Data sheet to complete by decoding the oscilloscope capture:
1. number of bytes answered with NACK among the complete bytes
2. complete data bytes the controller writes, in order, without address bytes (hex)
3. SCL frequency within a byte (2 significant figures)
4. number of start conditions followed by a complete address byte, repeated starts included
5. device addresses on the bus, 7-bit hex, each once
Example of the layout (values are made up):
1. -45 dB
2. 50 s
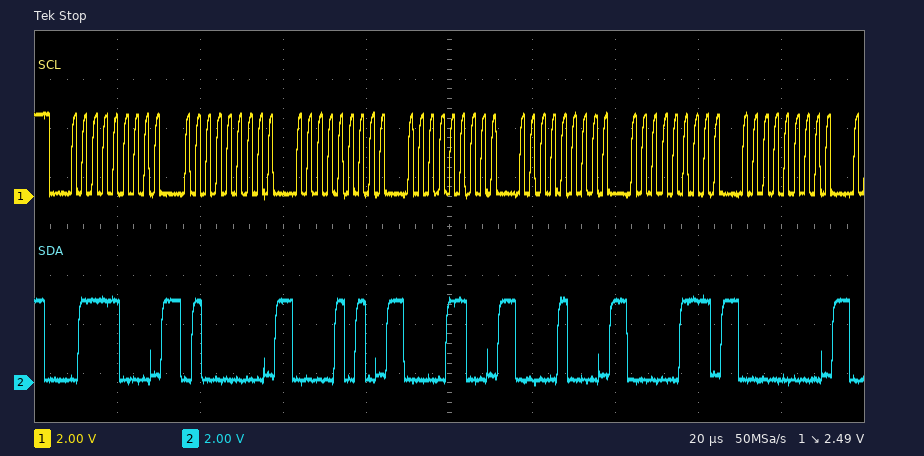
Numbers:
1. 0
2. 40 0A 0C 08 07 00
3. 400 kHz
4. 1
5. 0x3C
